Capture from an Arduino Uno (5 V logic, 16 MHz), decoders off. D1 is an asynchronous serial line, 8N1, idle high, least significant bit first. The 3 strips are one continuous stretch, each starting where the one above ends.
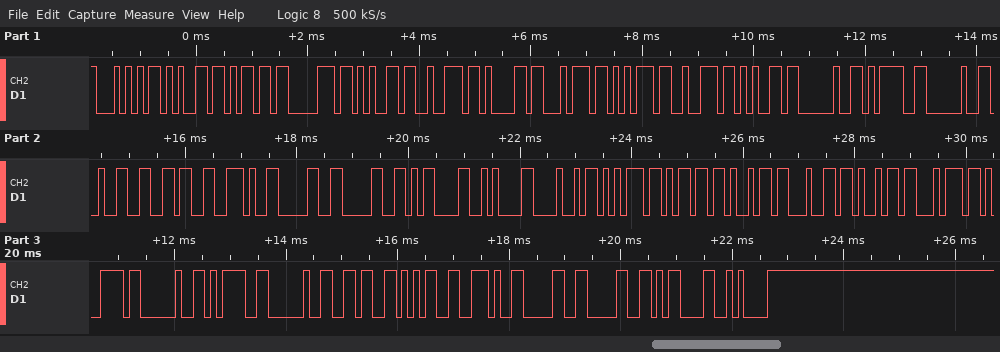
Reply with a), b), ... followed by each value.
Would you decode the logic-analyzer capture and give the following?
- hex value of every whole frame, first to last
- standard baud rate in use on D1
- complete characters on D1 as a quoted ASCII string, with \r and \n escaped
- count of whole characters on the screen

a) 54 65 6D 70 65 72 61 74 75 72 65 20 3D 20 32 36 2E 30 30 0D 0A 48 75 6D 69 64 69 74 79 20 3D 20 36 35 2E 30 30 0D 0A
b) 9600 baud
c) "Temperature = 26.00\r\nHumidity = 65.00\r\n"
d) 39
